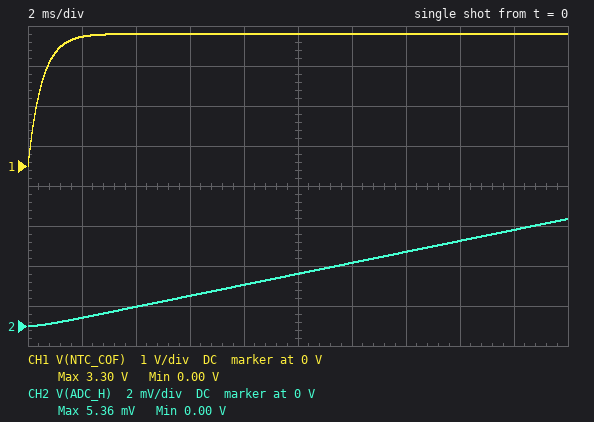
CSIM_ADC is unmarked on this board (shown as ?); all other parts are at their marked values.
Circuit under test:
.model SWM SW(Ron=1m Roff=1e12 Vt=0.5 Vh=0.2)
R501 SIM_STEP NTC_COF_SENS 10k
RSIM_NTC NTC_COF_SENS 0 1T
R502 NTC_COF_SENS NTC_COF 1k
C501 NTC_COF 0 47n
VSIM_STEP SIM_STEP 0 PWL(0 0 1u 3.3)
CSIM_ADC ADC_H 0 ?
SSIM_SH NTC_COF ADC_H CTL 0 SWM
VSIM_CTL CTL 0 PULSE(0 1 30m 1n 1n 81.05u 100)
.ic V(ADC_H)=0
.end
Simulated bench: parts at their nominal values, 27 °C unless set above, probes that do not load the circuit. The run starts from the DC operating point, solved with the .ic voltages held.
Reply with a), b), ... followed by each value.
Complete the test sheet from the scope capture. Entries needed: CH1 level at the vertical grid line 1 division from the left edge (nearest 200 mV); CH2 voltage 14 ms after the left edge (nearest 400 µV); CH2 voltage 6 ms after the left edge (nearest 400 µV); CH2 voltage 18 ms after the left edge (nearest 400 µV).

a) 3.2 V
b) 3.6 mV
c) 1.6 mV
d) 4.8 mV
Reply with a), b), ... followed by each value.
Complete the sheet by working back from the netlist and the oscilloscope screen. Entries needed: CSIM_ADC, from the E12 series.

a) 12 pF
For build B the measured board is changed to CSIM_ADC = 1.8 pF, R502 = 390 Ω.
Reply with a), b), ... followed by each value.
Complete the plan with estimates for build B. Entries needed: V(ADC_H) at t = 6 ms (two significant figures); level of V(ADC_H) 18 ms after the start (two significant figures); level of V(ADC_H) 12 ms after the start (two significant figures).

a) 10 mV
b) 32 mV
c) 21 mV
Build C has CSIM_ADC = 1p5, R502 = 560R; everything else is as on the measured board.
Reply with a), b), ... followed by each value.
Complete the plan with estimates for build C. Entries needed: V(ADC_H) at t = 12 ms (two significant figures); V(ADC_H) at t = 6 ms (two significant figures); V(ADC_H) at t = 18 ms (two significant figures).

a) 25 mV
b) 12 mV
c) 38 mV
